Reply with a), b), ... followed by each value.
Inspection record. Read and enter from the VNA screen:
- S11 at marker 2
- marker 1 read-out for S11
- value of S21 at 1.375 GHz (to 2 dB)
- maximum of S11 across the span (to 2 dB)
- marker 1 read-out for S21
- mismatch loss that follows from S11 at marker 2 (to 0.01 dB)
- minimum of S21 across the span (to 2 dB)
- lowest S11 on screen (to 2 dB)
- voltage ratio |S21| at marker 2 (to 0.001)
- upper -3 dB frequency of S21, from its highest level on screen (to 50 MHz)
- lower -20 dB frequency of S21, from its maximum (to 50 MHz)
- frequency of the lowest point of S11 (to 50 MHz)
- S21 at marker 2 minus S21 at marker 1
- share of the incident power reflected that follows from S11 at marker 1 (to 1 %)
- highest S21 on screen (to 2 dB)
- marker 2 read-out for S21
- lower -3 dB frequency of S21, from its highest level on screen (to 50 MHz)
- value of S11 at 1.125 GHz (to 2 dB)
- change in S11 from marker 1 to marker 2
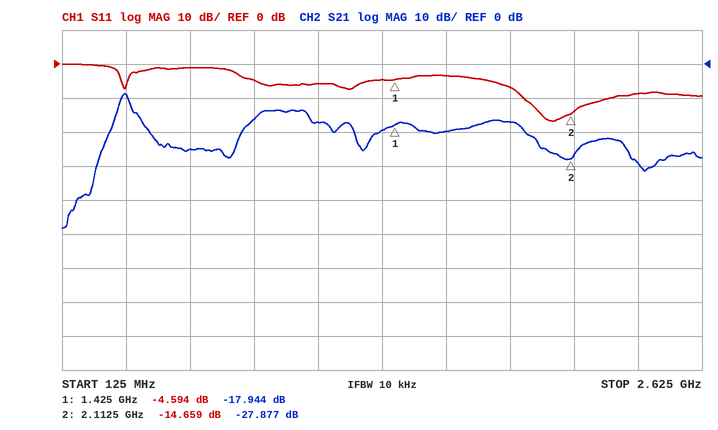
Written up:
a) -14.659 dB
b) -4.594 dB
c) -20 dB
d) 0 dB
e) -17.944 dB
f) 0.15 dB
g) -48 dB
h) -16 dB
i) 0.040
j) 400 MHz
k) 250 MHz
l) 2.05 GHz
m) -9.933 dB
n) 35 %
o) -8 dB
p) -27.877 dB
q) 350 MHz
r) -6 dB
s) -10.065 dB
